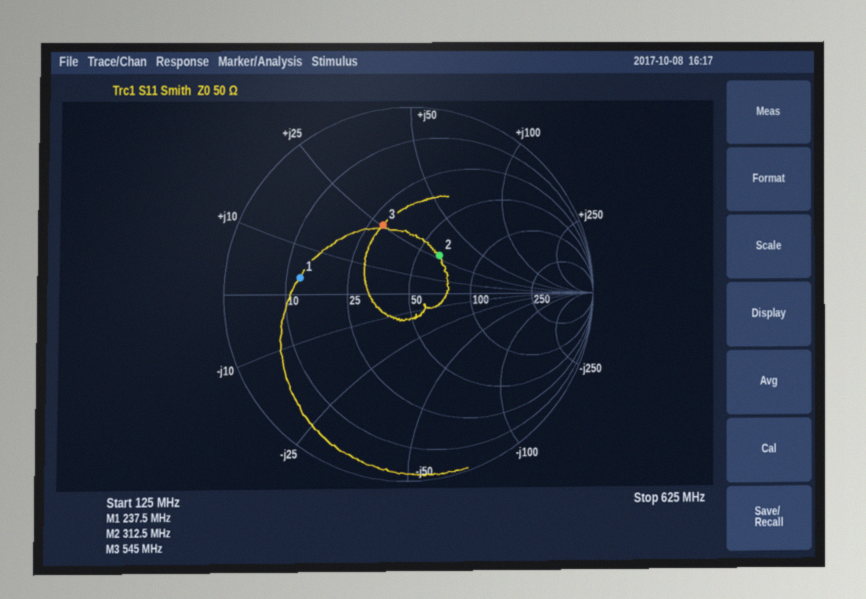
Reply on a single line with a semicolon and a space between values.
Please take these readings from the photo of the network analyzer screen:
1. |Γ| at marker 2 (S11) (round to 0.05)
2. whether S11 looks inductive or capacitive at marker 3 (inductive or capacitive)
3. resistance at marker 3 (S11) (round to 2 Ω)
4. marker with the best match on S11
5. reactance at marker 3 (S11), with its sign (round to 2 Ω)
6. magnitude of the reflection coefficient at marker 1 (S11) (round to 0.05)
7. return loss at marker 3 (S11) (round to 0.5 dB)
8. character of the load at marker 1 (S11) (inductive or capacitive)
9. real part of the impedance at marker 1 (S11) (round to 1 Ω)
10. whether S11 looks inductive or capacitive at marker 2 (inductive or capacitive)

0.25; inductive; 30 Ω; marker 2; +26 Ω; 0.60; 8.0 dB; inductive; 13 Ω; inductive
